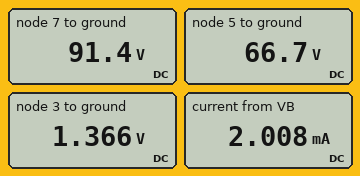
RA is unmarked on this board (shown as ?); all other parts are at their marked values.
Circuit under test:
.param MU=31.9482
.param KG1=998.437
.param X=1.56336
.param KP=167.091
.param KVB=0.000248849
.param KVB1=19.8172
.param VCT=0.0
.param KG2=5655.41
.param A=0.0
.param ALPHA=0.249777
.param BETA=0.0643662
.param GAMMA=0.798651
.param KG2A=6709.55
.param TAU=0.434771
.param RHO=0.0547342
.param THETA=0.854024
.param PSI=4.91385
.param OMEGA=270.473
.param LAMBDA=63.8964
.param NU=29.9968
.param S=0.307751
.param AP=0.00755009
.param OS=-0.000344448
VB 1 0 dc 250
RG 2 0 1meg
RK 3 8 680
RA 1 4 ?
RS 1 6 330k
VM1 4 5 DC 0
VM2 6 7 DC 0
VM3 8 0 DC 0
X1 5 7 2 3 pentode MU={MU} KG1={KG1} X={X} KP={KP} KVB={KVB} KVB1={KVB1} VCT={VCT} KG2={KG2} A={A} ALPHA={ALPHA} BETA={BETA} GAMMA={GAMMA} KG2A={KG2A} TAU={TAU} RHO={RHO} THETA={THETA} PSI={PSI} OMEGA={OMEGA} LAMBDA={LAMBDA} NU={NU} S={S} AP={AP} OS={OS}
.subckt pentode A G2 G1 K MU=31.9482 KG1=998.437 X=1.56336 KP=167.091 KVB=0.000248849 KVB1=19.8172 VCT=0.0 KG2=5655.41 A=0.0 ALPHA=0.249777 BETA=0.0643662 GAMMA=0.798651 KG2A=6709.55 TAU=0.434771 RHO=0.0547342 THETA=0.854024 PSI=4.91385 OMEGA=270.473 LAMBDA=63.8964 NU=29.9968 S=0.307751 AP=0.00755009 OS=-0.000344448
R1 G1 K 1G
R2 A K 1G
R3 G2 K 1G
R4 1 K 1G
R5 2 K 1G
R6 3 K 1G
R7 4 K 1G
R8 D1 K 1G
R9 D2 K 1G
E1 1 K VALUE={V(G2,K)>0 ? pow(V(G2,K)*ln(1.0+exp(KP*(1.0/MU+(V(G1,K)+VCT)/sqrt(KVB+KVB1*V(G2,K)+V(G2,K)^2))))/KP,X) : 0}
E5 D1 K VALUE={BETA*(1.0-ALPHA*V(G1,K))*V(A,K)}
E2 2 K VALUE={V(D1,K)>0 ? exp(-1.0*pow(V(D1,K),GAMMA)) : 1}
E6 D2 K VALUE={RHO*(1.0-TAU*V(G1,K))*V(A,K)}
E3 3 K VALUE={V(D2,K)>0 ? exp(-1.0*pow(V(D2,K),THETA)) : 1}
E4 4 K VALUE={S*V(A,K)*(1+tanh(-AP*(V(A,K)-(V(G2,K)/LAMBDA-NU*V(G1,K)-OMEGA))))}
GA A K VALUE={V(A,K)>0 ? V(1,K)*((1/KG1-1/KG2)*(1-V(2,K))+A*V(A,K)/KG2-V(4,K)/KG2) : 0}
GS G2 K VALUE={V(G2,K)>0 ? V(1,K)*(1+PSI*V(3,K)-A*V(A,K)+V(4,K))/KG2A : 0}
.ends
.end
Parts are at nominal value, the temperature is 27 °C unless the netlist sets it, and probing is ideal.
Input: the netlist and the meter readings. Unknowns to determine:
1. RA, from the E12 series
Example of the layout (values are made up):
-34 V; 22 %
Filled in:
120 kΩ
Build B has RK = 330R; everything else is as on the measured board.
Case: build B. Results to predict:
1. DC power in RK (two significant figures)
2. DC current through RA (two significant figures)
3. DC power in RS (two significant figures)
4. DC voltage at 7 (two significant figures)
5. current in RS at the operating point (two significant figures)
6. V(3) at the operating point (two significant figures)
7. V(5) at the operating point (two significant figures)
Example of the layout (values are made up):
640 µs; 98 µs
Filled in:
1.6 mW; 1.6 mA; 93 mW; 75 V; 530 µA; 720 mV; 53 V
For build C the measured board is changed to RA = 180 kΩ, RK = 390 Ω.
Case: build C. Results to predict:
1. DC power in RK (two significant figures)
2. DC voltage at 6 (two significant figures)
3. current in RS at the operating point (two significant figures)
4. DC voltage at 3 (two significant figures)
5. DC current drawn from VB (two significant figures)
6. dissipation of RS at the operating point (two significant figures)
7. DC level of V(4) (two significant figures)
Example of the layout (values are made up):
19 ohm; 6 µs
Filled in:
1.2 mW; 67 V; 550 µA; 690 mV; 1.8 mA; 100 mW; 31 V
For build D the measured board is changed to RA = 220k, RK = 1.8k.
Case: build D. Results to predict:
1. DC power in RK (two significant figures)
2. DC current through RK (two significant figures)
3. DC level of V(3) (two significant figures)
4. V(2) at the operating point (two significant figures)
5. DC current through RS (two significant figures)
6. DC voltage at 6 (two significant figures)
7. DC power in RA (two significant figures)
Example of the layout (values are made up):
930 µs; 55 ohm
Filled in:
3.5 mW; 1.4 mA; 2.5 V; 2.5 mV; 410 µA; 110 V; 210 mW
